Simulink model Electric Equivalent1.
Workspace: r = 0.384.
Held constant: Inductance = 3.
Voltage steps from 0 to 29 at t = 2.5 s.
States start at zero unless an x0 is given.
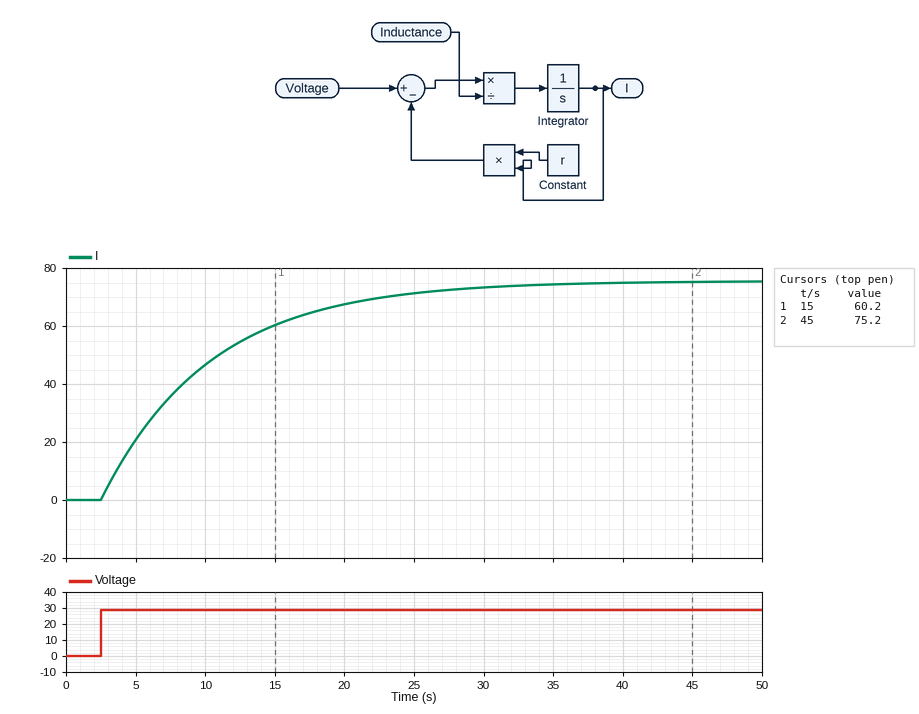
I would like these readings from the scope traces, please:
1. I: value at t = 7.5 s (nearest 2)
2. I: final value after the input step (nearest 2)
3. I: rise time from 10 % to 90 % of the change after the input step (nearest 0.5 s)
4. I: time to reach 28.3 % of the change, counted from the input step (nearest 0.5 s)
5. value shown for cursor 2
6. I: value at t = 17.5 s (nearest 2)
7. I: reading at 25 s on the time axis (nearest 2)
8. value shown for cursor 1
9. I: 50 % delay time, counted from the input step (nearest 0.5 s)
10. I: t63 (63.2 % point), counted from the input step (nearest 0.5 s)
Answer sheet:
36
76
17.0 s
2.5 s
75.2
64
72
60.2
5.5 s
8.0 s
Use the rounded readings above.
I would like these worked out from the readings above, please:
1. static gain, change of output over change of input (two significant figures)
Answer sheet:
2.6
